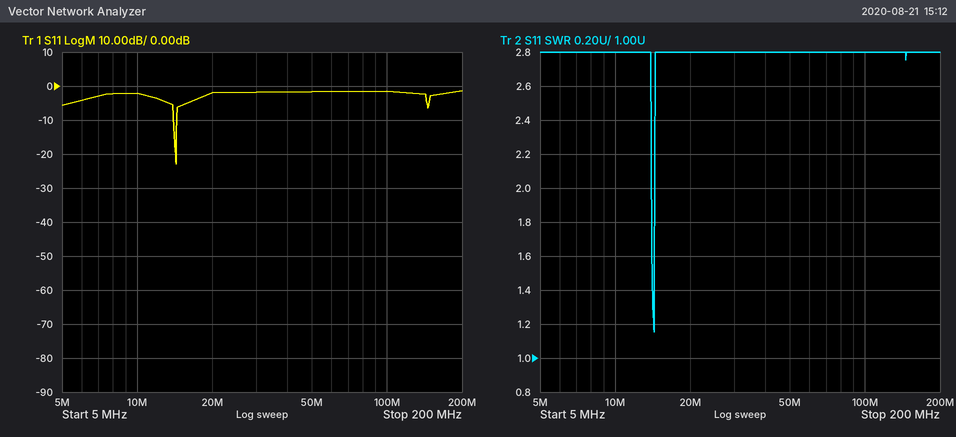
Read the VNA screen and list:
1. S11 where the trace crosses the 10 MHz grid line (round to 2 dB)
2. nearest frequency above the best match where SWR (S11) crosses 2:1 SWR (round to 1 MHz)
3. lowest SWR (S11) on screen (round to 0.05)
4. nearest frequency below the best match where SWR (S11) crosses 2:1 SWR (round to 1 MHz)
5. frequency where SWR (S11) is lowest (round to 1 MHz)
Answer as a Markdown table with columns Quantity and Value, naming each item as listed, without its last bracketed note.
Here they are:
| Quantity | Value |
|---|---|
| S11 where the trace crosses the 10 MHz grid line | -2 dB |
| nearest frequency above the best match where SWR (S11) crosses 2:1 SWR | 14 MHz |
| lowest SWR (S11) on screen | 1.15 |
| nearest frequency below the best match where SWR (S11) crosses 2:1 SWR | 14 MHz |
| frequency where SWR (S11) is lowest | 14 MHz |
